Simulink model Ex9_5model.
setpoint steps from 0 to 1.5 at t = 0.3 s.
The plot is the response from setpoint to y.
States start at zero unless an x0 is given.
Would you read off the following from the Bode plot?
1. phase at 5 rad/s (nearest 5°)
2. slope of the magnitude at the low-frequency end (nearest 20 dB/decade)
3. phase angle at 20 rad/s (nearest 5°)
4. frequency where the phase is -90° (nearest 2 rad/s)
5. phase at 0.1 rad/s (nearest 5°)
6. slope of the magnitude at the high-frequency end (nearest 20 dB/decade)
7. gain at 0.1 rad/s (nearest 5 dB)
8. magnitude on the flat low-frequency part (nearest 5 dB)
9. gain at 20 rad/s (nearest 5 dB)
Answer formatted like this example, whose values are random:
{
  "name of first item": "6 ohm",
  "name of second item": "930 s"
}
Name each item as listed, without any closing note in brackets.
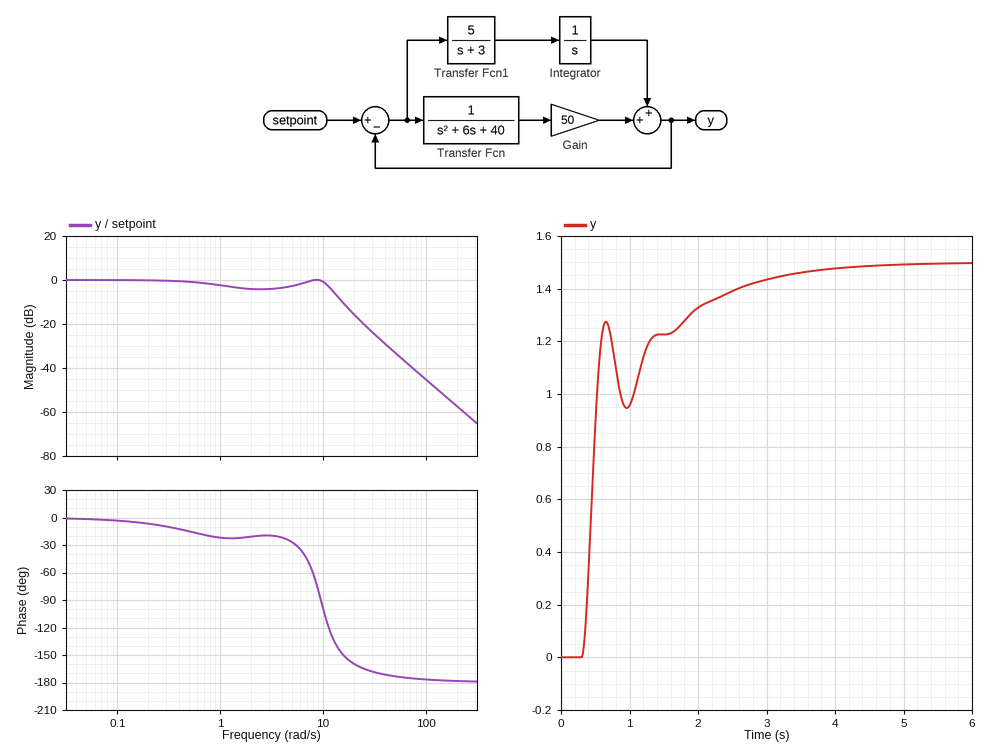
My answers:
{
  "phase at 5 rad/s": "-25°",
  "slope of the magnitude at the low-frequency end": "0 dB/decade",
  "phase angle at 20 rad/s": "-160°",
  "frequency where the phase is -90°": "10 rad/s",
  "phase at 0.1 rad/s": "-5°",
  "slope of the magnitude at the high-frequency end": "-40 dB/decade",
  "gain at 0.1 rad/s": "0 dB",
  "magnitude on the flat low-frequency part": "0 dB",
  "gain at 20 rad/s": "-15 dB"
}
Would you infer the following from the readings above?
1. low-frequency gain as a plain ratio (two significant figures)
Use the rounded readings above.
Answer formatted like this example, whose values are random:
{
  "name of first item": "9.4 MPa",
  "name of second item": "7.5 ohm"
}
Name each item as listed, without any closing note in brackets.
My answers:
{
  "low-frequency gain as a plain ratio": "1.0"
}
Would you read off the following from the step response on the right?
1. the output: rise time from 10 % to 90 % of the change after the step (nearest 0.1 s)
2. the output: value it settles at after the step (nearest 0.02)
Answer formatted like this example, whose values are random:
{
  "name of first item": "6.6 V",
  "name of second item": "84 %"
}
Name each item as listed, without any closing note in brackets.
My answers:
{
  "the output: rise time from 10 % to 90 % of the change after the step": "1.8 s",
  "the output: value it settles at after the step": "1.50"
}
